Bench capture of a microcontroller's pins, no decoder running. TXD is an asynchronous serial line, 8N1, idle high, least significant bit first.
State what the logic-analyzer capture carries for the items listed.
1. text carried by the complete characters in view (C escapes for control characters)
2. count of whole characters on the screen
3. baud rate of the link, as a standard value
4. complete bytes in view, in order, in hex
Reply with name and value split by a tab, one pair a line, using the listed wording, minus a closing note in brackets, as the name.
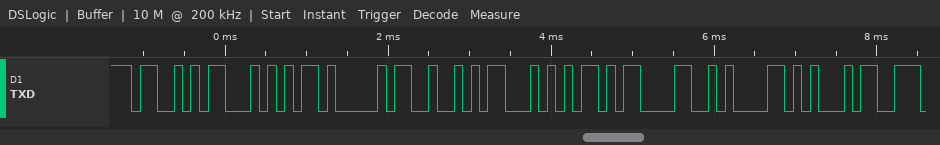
text carried by the complete characters in view	"START\r\nE"
count of whole characters on the screen	8
baud rate of the link, as a standard value	9600 baud
complete bytes in view, in order, in hex	0x53 0x54 0x41 0x52 0x54 0x0D 0x0A 0x45
